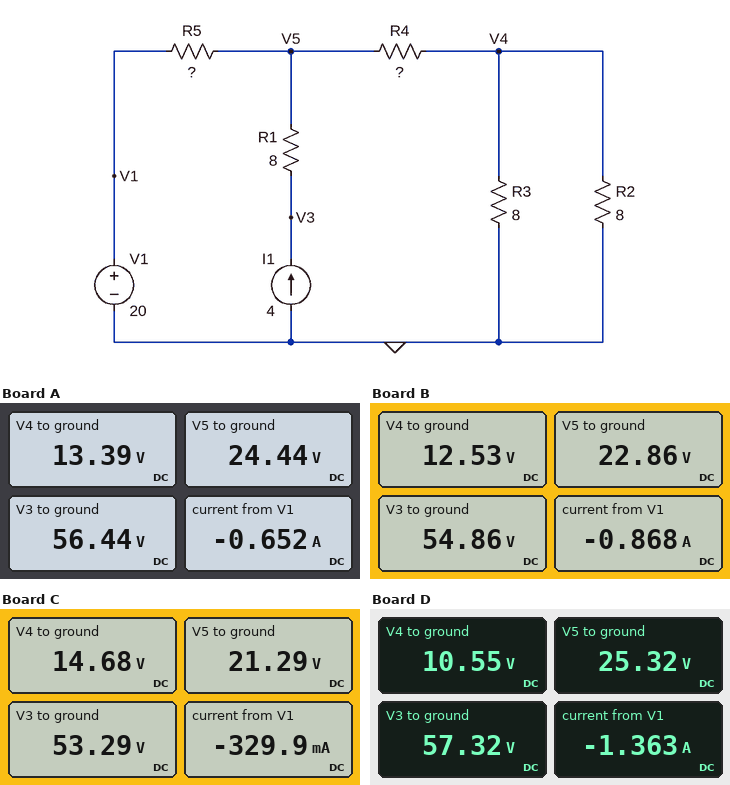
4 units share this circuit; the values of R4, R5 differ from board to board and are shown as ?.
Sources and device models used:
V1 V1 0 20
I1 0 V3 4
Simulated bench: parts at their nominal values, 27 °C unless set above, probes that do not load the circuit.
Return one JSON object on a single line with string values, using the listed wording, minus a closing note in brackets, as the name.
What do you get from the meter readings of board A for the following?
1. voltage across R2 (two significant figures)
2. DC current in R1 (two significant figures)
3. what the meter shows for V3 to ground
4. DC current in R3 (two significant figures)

{"voltage across R2": "13 V", "DC current in R1": "4.0 A", "what the meter shows for V3 to ground": "56.44 V", "DC current in R3": "1.7 A"}
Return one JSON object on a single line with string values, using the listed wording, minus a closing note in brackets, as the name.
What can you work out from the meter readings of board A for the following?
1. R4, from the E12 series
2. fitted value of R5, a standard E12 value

{"R4, from the E12 series": "3.3 Ω", "fitted value of R5, a standard E12 value": "6.8 Ω"}
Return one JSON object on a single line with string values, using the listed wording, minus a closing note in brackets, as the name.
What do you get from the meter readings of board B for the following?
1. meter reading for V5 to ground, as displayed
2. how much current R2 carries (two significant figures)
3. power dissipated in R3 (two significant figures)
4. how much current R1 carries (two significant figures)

{"meter reading for V5 to ground, as displayed": "22.86 V", "how much current R2 carries": "1.6 A", "power dissipated in R3": "20 W", "how much current R1 carries": "4.0 A"}
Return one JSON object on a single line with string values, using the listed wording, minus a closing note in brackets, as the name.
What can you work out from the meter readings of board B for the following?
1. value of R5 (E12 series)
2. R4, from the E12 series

{"value of R5": "3.3 Ω", "R4, from the E12 series": "3.3 Ω"}
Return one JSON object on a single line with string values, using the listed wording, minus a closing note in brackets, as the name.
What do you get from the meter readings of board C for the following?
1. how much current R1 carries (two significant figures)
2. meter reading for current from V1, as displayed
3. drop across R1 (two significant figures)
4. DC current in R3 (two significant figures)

{"how much current R1 carries": "4.0 A", "meter reading for current from V1, as displayed": "-329.9 mA", "drop across R1": "32 V", "DC current in R3": "1.8 A"}
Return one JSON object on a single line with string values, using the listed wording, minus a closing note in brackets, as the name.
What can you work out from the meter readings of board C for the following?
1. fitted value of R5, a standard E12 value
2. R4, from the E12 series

{"fitted value of R5, a standard E12 value": "3.9 Ω", "R4, from the E12 series": "1.8 Ω"}
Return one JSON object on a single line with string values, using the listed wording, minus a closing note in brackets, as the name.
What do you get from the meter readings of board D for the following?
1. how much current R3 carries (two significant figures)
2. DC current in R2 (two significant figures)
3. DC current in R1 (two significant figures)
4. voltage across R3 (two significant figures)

{"how much current R3 carries": "1.3 A", "DC current in R2": "1.3 A", "DC current in R1": "4.0 A", "voltage across R3": "11 V"}
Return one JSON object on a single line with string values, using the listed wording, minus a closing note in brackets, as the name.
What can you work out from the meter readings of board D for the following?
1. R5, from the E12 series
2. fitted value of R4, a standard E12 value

{"R5, from the E12 series": "3.9 Ω", "fitted value of R4, a standard E12 value": "5.6 Ω"}
